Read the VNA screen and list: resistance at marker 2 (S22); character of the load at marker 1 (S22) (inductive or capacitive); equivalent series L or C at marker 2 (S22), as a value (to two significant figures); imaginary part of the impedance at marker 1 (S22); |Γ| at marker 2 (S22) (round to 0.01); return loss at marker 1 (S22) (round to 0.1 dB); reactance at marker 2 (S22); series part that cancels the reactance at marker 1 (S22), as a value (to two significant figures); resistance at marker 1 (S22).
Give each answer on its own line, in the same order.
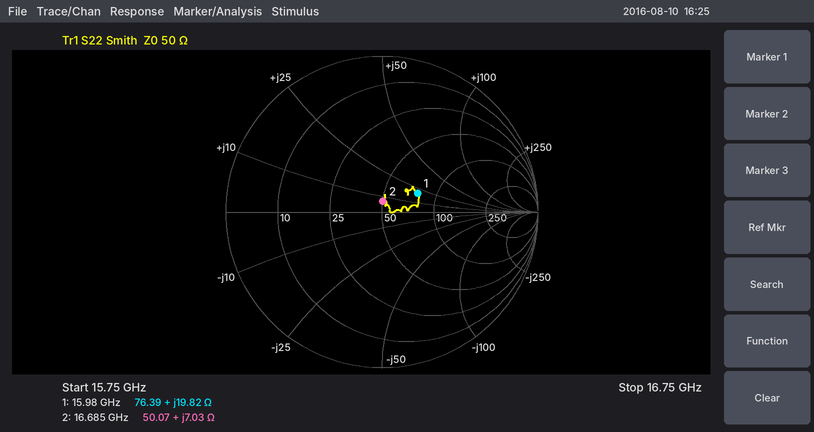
50.07 Ω
inductive
67 pH
+19.82 Ω
0.07
11.8 dB
+7.03 Ω
500 fF
76.39 Ω
